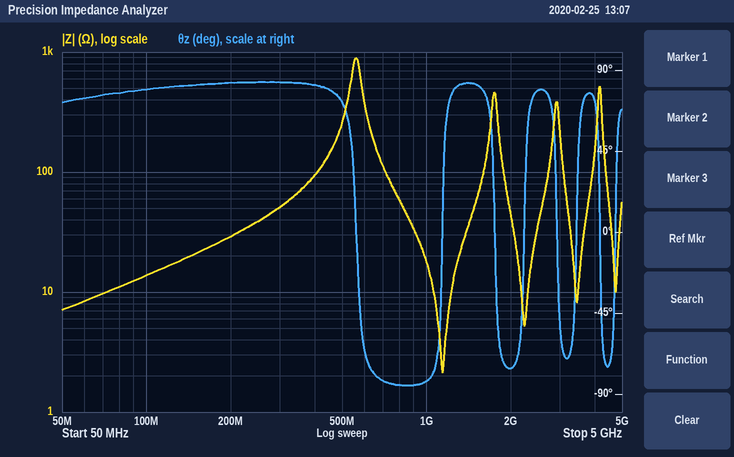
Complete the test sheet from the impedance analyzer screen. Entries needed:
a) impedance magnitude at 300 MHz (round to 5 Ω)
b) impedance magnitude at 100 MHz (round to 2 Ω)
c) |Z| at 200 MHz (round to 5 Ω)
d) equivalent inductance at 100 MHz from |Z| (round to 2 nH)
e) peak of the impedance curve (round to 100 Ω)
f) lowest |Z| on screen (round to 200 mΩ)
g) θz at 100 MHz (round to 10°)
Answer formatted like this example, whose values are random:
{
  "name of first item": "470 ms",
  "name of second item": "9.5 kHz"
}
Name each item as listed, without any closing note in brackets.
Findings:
{
  "impedance magnitude at 300 MHz": "50 Ω",
  "impedance magnitude at 100 MHz": "14 Ω",
  "|Z| at 200 MHz": "30 Ω",
  "equivalent inductance at 100 MHz from |Z|": "22 nH",
  "peak of the impedance curve": "900 Ω",
  "lowest |Z| on screen": "2.2 Ω",
  "θz at 100 MHz": "80°"
}
